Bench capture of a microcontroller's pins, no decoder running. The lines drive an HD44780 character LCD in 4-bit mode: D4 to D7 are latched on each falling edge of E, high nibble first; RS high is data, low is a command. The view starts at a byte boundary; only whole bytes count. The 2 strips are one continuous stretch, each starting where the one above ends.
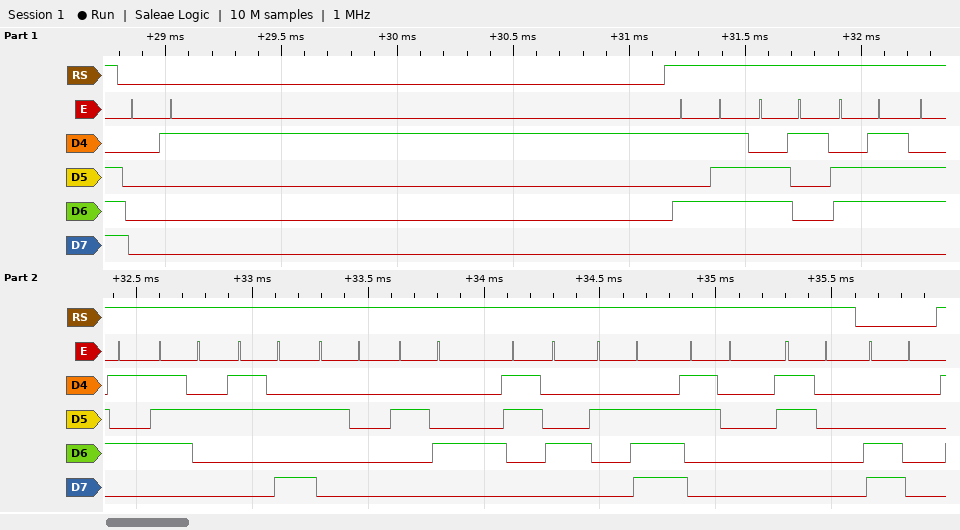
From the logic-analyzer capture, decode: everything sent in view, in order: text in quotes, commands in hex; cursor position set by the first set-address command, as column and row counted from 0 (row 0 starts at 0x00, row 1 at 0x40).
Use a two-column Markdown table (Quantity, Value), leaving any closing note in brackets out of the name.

| Quantity | Value |
|---|---|
| everything sent in view, in order: text in quotes, commands in hex | 0x01 "Wager: $4.00" 0xC0 |
| cursor position set by the first set-address command, as column and row counted from 0 | column 0, row 1 |
